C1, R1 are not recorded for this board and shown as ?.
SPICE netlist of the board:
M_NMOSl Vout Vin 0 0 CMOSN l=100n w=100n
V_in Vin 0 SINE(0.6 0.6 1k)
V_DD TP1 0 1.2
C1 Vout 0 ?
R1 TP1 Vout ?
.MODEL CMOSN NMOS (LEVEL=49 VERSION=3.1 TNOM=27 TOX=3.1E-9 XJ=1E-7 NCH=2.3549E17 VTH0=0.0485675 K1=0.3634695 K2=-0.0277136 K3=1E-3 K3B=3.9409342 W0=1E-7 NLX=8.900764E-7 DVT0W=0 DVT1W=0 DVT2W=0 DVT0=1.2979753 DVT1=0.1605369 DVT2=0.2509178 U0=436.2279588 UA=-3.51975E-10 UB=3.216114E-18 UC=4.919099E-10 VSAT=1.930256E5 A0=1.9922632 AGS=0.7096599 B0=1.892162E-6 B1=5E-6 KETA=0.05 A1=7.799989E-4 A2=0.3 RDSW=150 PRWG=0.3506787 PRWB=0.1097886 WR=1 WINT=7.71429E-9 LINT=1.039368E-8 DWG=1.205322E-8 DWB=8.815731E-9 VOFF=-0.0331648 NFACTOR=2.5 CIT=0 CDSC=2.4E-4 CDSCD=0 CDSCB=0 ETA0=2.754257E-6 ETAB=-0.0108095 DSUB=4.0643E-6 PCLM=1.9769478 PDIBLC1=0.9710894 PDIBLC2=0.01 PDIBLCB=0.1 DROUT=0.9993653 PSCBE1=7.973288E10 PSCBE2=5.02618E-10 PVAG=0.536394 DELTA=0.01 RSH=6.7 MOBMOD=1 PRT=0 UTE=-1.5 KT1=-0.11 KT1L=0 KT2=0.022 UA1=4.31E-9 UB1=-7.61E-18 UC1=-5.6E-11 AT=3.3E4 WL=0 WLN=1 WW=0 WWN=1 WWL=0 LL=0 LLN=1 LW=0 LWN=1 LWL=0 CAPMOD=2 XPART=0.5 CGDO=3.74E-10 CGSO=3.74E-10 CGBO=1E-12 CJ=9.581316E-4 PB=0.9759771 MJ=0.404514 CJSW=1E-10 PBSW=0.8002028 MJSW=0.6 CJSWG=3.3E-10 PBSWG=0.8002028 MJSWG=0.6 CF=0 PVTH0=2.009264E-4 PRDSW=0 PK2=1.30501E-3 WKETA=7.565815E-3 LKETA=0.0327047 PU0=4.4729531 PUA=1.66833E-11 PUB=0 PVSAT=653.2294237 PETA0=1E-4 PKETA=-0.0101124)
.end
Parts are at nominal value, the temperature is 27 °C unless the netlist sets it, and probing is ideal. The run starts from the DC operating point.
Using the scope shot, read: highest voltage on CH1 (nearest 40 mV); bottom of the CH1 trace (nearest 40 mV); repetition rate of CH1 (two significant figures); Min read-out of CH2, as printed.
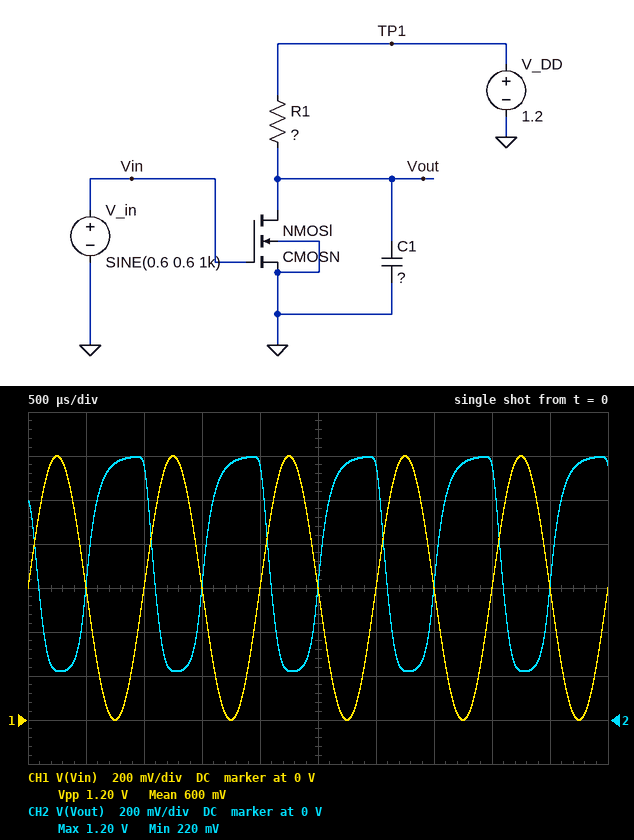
1.20 V
0 V
1.0 kHz
220 mV
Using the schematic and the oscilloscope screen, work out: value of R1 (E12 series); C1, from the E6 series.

39 kΩ
2.2 nF
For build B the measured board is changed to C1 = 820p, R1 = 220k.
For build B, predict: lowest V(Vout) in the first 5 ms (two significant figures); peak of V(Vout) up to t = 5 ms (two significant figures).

38 mV
1.1 V
